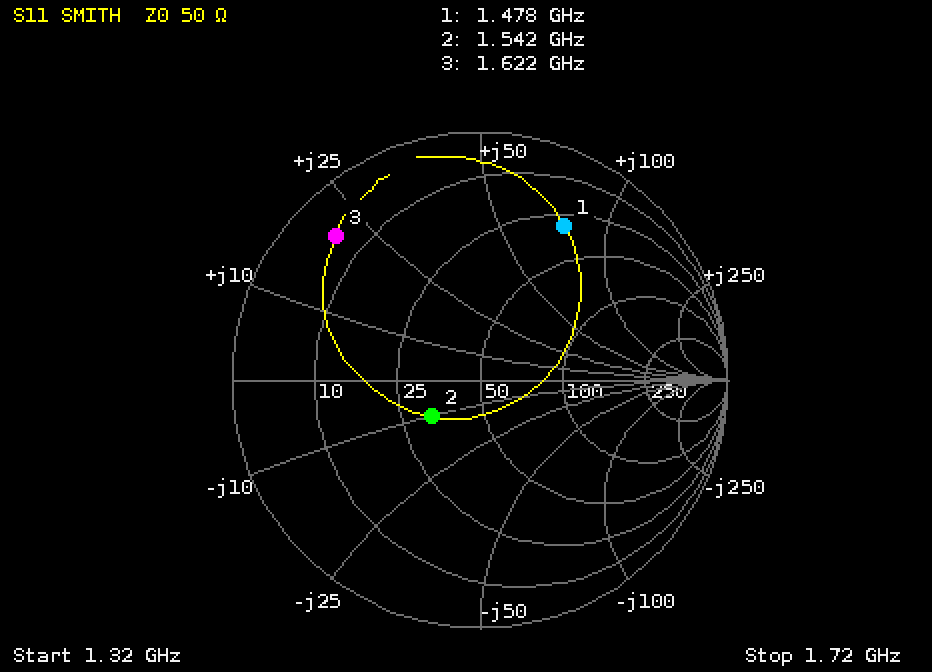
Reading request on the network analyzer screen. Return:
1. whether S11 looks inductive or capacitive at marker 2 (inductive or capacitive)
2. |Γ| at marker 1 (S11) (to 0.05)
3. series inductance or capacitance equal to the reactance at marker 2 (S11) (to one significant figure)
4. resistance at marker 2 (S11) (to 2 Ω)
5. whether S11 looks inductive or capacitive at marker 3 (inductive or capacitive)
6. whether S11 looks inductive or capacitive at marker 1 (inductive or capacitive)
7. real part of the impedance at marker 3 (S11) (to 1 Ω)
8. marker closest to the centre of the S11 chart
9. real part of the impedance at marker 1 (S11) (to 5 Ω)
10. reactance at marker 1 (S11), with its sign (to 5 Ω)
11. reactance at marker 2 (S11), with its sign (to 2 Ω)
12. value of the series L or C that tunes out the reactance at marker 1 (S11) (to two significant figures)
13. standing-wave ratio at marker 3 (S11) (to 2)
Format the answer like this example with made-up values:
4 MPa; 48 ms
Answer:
capacitive; 0.70; 10 pF; 32 Ω; inductive; inductive; 6 Ω; marker 2; 30 Ω; +75 Ω; -10 Ω; 1.4 pF; 10
